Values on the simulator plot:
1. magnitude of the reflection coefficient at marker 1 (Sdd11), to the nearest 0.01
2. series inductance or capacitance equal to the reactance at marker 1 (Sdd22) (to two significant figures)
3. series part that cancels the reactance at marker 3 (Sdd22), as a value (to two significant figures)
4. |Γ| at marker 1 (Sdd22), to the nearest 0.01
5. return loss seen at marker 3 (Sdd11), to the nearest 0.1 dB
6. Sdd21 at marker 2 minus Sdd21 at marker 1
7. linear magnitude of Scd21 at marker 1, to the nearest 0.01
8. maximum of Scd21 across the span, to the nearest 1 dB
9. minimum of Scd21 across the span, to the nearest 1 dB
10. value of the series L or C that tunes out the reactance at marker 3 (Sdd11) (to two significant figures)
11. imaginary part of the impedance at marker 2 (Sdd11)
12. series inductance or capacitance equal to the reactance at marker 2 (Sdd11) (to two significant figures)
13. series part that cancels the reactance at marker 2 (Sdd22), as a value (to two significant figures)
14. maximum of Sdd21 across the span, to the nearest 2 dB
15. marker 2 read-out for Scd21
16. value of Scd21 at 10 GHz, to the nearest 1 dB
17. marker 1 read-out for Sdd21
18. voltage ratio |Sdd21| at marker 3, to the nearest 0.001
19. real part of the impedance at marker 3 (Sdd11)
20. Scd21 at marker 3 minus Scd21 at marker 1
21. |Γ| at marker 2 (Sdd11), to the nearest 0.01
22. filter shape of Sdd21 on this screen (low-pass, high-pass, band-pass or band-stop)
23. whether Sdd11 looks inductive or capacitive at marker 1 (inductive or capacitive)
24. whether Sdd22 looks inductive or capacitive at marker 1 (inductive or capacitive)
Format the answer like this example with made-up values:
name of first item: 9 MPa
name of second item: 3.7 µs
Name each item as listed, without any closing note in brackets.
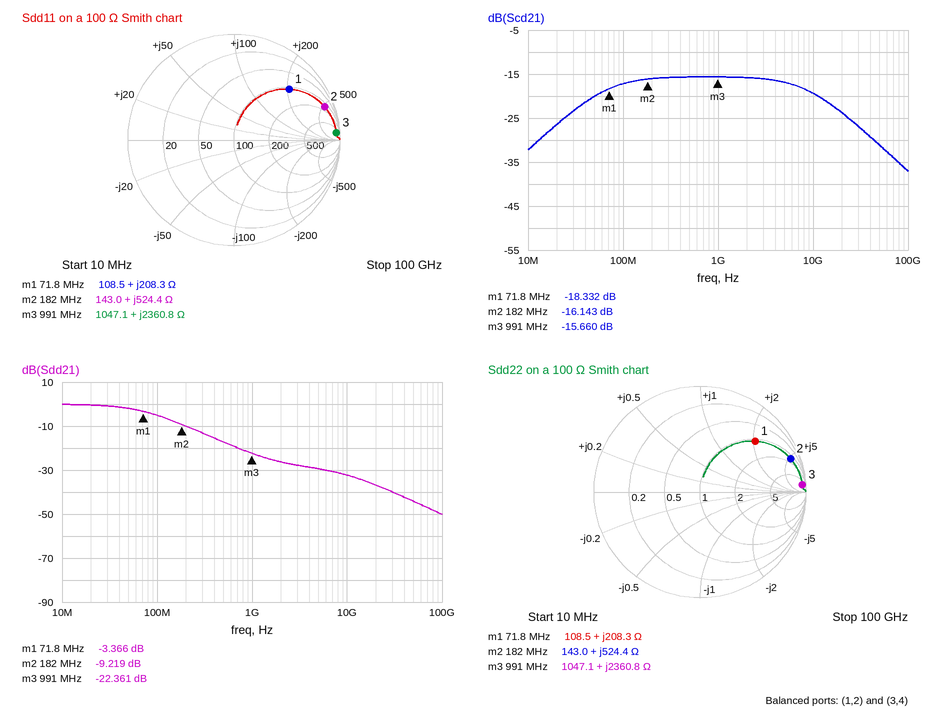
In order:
magnitude of the reflection coefficient at marker 1 (Sdd11), to the nearest 0.01: 0.71
series inductance or capacitance equal to the reactance at marker 1 (Sdd22): 460 nH
series part that cancels the reactance at marker 3 (Sdd22), as a value: 68 fF
|Γ| at marker 1 (Sdd22), to the nearest 0.01: 0.71
return loss seen at marker 3 (Sdd11), to the nearest 0.1 dB: 0.3 dB
Sdd21 at marker 2 minus Sdd21 at marker 1: -5.853 dB
linear magnitude of Scd21 at marker 1, to the nearest 0.01: 0.12
maximum of Scd21 across the span, to the nearest 1 dB: -16 dB
minimum of Scd21 across the span, to the nearest 1 dB: -37 dB
value of the series L or C that tunes out the reactance at marker 3 (Sdd11): 68 fF
imaginary part of the impedance at marker 2: +524.4 Ω
series inductance or capacitance equal to the reactance at marker 2 (Sdd11): 460 nH
series part that cancels the reactance at marker 2 (Sdd22), as a value: 1.7 pF
maximum of Sdd21 across the span, to the nearest 2 dB: 0 dB
marker 2 read-out for Scd21: -16.143 dB
value of Scd21 at 10 GHz, to the nearest 1 dB: -19 dB
marker 1 read-out for Sdd21: -3.366 dB
voltage ratio |Sdd21| at marker 3, to the nearest 0.001: 0.076
real part of the impedance at marker 3: 1047.1 Ω
Scd21 at marker 3 minus Scd21 at marker 1: 2.672 dB
|Γ| at marker 2 (Sdd11), to the nearest 0.01: 0.91
filter shape of Sdd21 on this screen: low-pass
whether Sdd11 looks inductive or capacitive at marker 1: inductive
whether Sdd22 looks inductive or capacitive at marker 1: inductive
